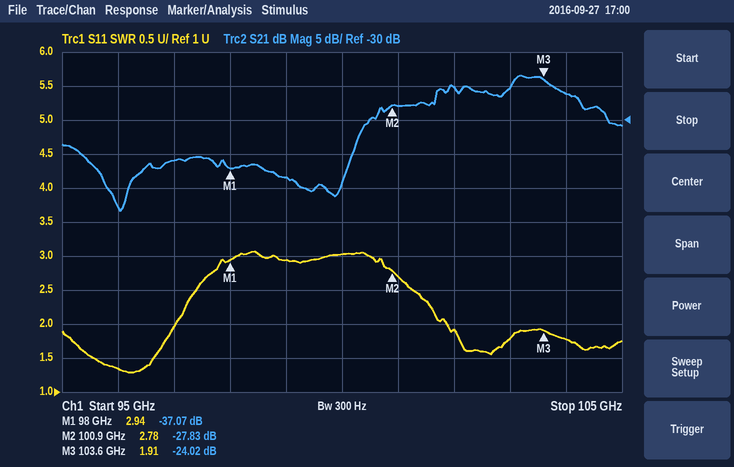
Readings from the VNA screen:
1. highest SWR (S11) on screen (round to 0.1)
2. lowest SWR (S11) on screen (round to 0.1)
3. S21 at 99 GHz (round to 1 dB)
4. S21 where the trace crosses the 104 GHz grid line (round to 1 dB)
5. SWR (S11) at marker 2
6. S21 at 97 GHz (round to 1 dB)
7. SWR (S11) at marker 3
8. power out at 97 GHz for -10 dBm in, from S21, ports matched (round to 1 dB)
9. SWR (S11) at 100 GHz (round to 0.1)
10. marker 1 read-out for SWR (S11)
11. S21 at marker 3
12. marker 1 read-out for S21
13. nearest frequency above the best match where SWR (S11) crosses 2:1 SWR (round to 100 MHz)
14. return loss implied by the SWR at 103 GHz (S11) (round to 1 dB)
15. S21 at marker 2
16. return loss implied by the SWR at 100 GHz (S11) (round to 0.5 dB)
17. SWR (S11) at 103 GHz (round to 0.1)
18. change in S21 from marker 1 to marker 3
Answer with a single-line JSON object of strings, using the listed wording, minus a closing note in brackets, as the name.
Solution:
{"highest SWR (S11) on screen": "3.1", "lowest SWR (S11) on screen": "1.3", "S21 at 99 GHz": "-38 dB", "S21 where the trace crosses the 104 GHz grid line": "-26 dB", "SWR (S11) at marker 2": "2.78", "S21 at 97 GHz": "-36 dB", "SWR (S11) at marker 3": "1.91", "power out at 97 GHz for -10 dBm in, from S21, ports matched": "-46 dBm", "SWR (S11) at 100 GHz": "3.0", "marker 1 read-out for SWR": "2.94", "S21 at marker 3": "-24.02 dB", "marker 1 read-out for S21": "-37.07 dB", "nearest frequency above the best match where SWR (S11) crosses 2:1 SWR": "97.0 GHz", "return loss implied by the SWR at 103 GHz (S11)": "11 dB", "S21 at marker 2": "-27.83 dB", "return loss implied by the SWR at 100 GHz (S11)": "6.0 dB", "SWR (S11) at 103 GHz": "1.8", "change in S21 from marker 1 to marker 3": "13.05 dB"}
